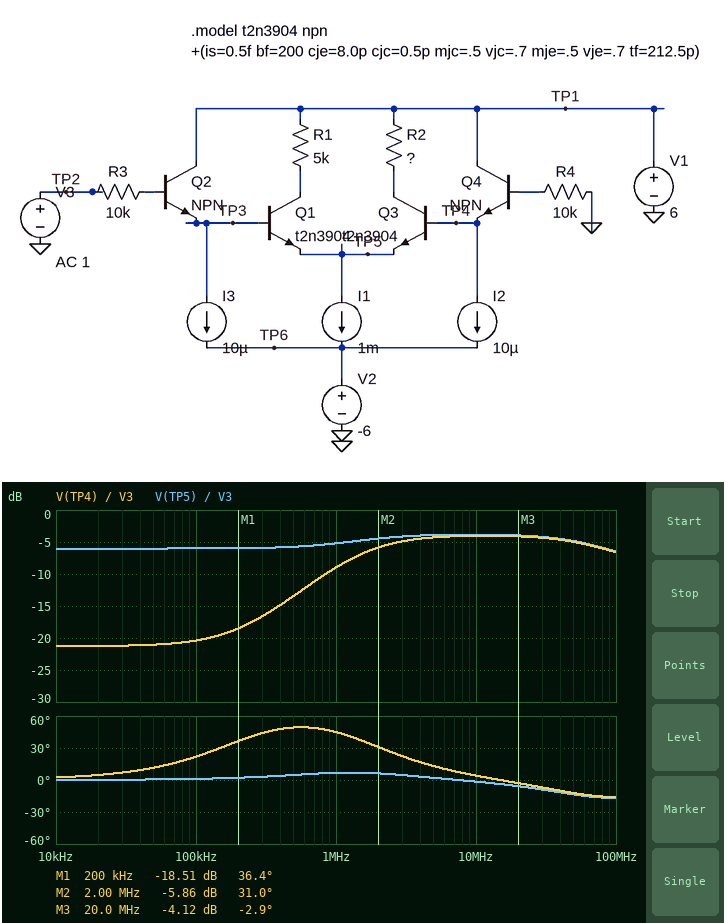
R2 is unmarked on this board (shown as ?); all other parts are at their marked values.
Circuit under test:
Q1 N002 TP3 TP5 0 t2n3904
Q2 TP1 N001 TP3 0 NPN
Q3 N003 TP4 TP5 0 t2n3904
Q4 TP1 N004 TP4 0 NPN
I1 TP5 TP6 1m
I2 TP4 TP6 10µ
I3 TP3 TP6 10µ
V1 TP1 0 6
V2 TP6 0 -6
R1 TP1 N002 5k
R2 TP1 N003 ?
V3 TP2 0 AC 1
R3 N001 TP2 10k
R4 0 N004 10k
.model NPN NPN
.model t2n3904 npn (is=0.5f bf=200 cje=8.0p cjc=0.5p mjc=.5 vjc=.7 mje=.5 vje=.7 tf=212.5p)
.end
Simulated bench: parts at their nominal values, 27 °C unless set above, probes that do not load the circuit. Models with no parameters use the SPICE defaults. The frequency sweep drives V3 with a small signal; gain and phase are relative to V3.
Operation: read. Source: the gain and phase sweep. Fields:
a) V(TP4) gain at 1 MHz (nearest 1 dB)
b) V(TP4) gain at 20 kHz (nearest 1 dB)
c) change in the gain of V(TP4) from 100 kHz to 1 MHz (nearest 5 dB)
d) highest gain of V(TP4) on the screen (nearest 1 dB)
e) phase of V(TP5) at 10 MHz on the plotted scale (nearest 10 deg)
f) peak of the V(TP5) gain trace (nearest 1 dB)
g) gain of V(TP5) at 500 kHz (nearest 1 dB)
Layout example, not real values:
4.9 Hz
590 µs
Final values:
-9 dB
-21 dB
10 dB
-4 dB
0 deg
-4 dB
-6 dB
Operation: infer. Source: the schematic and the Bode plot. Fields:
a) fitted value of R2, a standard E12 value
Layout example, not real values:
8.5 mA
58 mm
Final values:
10 kΩ
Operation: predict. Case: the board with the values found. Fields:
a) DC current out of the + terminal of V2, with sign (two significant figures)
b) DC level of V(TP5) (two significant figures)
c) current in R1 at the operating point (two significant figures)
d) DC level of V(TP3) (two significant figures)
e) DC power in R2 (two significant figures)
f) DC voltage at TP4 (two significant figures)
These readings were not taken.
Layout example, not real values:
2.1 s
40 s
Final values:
-1.0 mA
-1.4 V
500 µA
-660 mV
2.5 mW
-660 mV
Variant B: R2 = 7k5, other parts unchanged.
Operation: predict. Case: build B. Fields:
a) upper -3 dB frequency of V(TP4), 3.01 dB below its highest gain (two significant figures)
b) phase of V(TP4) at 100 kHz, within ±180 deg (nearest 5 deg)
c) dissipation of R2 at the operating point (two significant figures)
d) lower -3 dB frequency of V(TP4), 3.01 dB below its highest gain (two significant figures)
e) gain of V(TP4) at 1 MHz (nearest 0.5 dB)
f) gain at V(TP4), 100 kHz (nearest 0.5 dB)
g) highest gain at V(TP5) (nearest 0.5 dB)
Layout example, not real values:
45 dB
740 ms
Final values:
200 MHz
15 deg
1.9 mW
1.8 MHz
-11.0 dB
-21.0 dB
-5.0 dB
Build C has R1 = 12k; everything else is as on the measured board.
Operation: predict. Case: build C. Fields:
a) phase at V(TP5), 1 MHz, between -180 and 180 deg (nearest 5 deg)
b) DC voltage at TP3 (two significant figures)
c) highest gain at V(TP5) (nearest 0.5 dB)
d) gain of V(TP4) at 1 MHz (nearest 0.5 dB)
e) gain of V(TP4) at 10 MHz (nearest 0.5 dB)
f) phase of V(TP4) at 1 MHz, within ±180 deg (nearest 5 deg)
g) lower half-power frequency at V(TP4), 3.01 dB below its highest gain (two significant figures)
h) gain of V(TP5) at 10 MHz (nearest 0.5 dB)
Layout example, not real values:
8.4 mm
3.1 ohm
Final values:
-5 deg
-660 mV
-6.0 dB
-10.5 dB
-8.0 dB
35 deg
1.0 MHz
-7.5 dB
